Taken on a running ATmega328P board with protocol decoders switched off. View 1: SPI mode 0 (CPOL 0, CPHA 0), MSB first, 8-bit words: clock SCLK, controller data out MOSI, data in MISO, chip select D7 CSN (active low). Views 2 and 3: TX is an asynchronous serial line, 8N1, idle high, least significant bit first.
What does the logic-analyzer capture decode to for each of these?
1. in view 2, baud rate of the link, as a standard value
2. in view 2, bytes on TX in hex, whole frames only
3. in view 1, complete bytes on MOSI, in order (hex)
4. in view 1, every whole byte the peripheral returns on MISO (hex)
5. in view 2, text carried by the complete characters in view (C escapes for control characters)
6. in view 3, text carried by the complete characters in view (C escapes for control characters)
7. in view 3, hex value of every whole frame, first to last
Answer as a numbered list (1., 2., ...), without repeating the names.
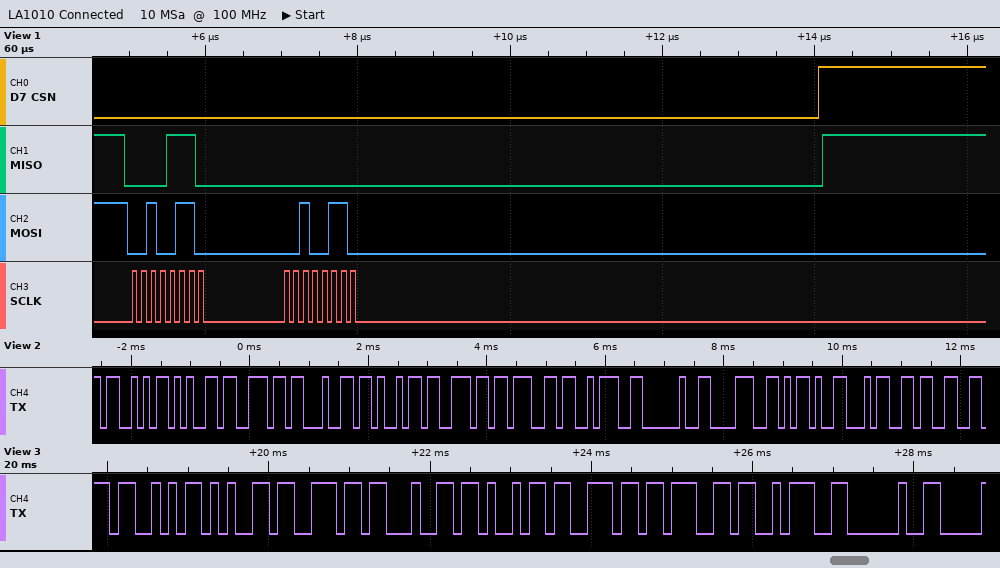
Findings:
1. 9600 baud
2. 0x53 0x65 0x6E 0x64 0x69 0x6E 0x67 0x3A 0x20 0x38 0x2D 0x34 0x33
3. 26 26
4. 0E 00
5. "Sending: 8-43"
6. "Sending: "
7. 53 65 6E 64 69 6E 67 3A 20
